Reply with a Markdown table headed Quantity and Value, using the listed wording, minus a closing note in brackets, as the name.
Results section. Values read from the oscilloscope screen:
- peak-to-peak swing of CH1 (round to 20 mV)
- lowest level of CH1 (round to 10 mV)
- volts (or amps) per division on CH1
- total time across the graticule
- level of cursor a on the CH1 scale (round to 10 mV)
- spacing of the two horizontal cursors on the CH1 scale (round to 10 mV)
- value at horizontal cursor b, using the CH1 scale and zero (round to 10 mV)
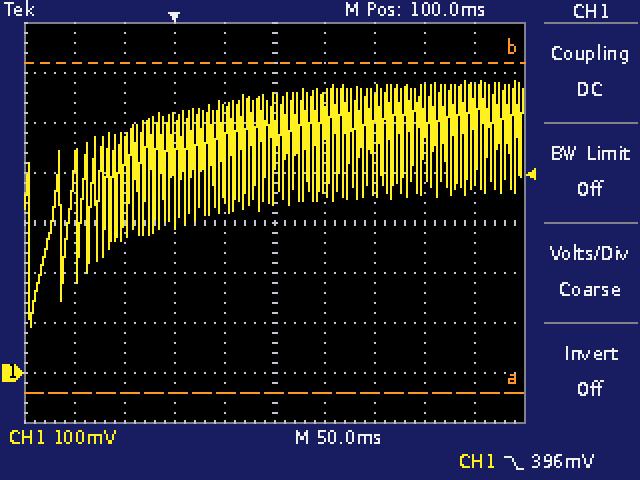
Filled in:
| Quantity | Value |
|---|---|
| peak-to-peak swing of CH1 | 500 mV |
| lowest level of CH1 | 90 mV |
| volts (or amps) per division on CH1 | 100 mV |
| total time across the graticule | 500 ms |
| level of cursor a on the CH1 scale | -40 mV |
| spacing of the two horizontal cursors on the CH1 scale | 660 mV |
| value at horizontal cursor b, using the CH1 scale and zero | 620 mV |
